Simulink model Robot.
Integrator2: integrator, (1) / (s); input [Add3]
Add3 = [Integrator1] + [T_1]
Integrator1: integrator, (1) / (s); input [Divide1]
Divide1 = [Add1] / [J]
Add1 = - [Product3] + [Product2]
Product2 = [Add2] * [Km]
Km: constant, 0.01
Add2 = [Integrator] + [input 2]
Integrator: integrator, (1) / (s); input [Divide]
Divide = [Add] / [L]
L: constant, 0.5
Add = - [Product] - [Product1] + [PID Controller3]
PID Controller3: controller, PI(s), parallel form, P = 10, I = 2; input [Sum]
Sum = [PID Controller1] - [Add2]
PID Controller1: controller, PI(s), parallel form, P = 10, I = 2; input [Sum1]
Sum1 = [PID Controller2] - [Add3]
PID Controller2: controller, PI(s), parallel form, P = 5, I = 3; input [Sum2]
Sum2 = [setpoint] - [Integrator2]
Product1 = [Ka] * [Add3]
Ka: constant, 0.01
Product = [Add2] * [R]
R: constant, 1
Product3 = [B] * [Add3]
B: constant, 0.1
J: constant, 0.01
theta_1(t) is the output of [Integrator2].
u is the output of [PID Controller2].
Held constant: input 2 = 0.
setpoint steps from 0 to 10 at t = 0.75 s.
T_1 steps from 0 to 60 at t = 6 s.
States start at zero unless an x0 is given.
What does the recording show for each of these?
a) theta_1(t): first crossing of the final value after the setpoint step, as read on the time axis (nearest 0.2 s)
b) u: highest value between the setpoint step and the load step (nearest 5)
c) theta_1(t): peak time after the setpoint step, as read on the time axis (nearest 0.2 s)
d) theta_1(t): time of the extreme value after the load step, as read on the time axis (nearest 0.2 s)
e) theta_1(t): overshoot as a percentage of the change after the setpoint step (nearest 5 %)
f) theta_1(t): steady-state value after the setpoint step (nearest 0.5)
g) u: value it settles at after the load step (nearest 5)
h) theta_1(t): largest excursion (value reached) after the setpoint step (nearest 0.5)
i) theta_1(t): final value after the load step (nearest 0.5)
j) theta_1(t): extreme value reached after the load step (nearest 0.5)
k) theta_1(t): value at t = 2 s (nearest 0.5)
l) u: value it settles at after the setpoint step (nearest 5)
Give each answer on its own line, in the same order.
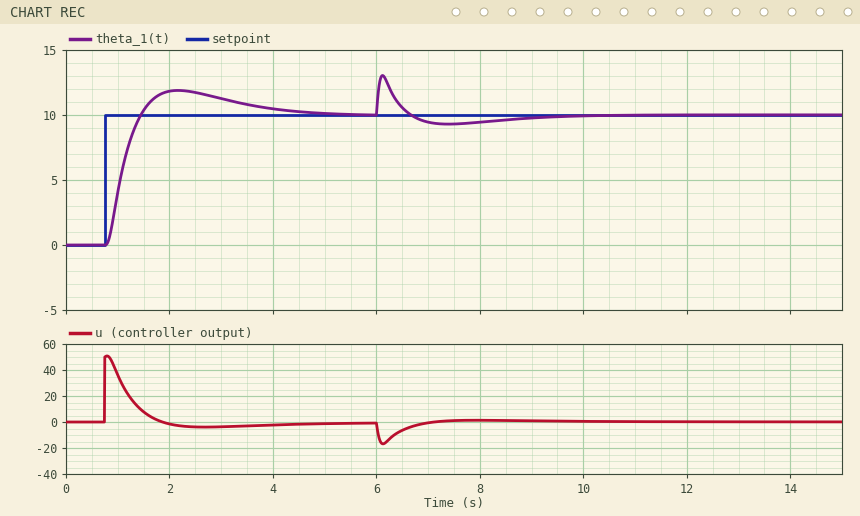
1.4 s
50
2.2 s
6.2 s
20 %
10.0
0
12.0
10.0
13.0
12.0
0
